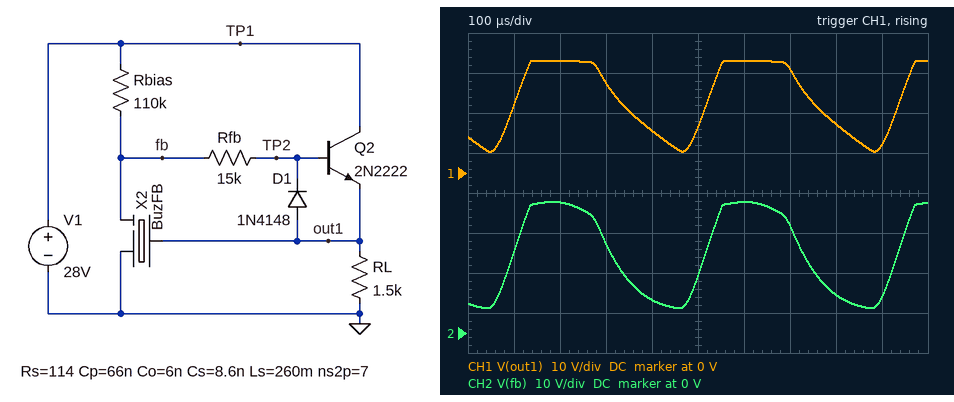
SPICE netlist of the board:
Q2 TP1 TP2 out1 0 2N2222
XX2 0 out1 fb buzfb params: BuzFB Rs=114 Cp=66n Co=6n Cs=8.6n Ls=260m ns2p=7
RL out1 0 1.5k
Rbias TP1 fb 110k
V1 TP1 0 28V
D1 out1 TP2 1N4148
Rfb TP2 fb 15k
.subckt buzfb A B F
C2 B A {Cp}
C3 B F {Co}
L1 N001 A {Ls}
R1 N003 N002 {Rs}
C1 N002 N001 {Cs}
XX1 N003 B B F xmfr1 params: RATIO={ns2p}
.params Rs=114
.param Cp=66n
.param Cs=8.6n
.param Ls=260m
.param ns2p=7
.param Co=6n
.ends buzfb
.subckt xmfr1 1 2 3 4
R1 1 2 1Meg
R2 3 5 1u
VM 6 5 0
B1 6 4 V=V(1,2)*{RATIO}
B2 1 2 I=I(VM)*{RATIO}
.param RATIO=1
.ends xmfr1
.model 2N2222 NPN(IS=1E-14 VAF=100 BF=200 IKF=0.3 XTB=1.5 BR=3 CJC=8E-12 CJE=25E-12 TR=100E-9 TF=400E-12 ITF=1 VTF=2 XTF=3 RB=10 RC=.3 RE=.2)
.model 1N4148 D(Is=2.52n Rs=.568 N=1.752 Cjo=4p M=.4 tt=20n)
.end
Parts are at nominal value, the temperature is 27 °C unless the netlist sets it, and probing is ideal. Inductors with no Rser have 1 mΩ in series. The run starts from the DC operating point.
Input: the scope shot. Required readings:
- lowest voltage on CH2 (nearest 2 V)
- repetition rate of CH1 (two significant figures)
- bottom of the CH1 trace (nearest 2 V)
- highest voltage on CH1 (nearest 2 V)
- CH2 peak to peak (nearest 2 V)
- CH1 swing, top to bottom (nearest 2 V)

6 V
2.4 kHz
6 V
28 V
26 V
22 V
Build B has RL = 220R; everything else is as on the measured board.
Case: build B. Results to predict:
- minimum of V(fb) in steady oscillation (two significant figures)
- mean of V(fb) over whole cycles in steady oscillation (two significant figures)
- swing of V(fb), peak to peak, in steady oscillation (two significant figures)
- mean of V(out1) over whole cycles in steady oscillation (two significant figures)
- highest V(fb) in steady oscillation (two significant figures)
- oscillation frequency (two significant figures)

-12 V
14 V
57 V
12 V
45 V
3.1 kHz
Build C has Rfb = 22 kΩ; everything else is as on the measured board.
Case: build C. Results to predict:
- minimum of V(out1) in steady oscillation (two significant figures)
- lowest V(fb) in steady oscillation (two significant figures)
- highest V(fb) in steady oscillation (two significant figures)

5.1 V
6.0 V
33 V
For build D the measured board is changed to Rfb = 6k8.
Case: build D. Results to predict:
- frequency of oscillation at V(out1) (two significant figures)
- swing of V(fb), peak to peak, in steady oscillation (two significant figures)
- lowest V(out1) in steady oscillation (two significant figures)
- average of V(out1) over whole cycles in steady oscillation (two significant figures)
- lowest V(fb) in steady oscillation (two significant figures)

3.0 kHz
25 V
7.4 V
21 V
8.3 V
